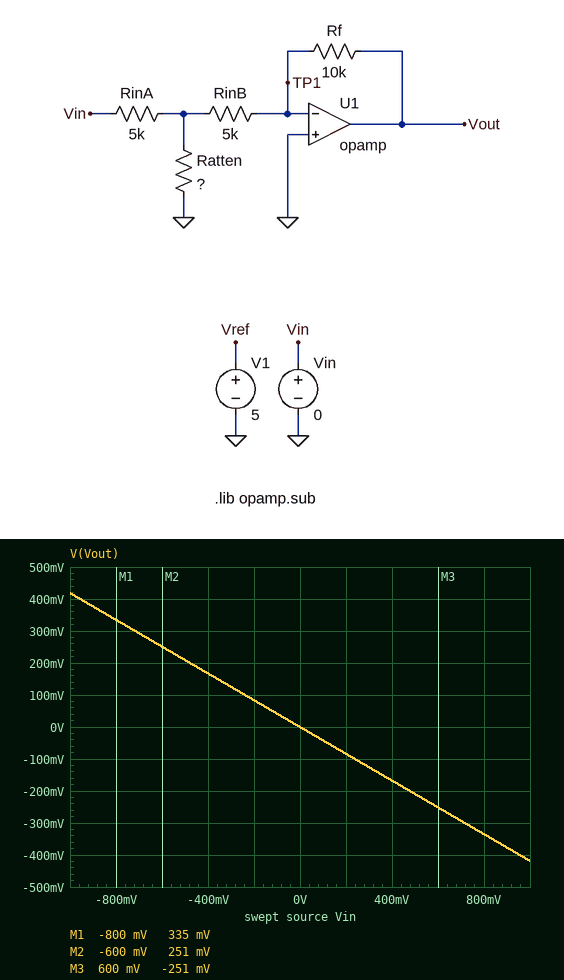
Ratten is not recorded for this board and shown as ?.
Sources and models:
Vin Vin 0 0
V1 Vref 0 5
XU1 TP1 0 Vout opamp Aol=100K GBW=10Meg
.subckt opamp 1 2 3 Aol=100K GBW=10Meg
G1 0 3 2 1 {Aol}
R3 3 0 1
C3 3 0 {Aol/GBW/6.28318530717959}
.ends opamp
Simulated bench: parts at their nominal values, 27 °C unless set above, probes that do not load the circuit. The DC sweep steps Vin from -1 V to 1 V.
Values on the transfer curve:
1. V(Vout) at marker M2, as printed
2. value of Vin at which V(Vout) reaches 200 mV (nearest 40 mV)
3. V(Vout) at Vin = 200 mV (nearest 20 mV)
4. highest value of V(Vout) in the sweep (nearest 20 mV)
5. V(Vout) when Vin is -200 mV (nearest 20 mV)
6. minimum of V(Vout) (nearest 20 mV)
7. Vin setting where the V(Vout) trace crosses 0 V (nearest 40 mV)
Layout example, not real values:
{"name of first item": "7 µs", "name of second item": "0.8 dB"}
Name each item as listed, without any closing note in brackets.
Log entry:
{"V(Vout) at marker M2, as printed": "251 mV", "value of Vin at which V(Vout) reaches 200 mV": "-480 mV", "V(Vout) at Vin = 200 mV": "-80 mV", "highest value of V(Vout) in the sweep": "420 mV", "V(Vout) when Vin is -200 mV": "80 mV", "minimum of V(Vout)": "-420 mV", "Vin setting where the V(Vout) trace crosses 0 V": "0 V"}
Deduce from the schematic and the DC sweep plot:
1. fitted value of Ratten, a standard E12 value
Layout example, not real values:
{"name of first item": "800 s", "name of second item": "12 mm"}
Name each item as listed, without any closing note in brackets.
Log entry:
{"fitted value of Ratten, a standard E12 value": "1.8 kΩ"}
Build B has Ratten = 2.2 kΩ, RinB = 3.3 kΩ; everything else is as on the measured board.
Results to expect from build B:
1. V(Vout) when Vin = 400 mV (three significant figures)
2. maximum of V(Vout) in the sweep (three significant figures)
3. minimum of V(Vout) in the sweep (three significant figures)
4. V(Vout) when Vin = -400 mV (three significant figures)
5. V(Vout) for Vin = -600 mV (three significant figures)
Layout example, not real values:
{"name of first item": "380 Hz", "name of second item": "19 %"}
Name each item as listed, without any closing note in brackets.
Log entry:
{"V(Vout) when Vin = 400 mV": "-253 mV", "maximum of V(Vout) in the sweep": "633 mV", "minimum of V(Vout) in the sweep": "-633 mV", "V(Vout) when Vin = -400 mV": "253 mV", "V(Vout) for Vin = -600 mV": "380 mV"}
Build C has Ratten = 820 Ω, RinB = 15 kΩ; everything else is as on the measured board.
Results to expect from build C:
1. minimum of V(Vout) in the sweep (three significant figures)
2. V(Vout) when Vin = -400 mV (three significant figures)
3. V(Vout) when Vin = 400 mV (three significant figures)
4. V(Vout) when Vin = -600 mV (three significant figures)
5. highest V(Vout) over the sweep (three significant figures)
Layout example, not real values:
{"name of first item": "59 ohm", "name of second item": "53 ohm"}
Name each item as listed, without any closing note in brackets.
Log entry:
{"minimum of V(Vout) in the sweep": "-89.7 mV", "V(Vout) when Vin = -400 mV": "35.9 mV", "V(Vout) when Vin = 400 mV": "-35.9 mV", "V(Vout) when Vin = -600 mV": "53.8 mV", "highest V(Vout) over the sweep": "89.7 mV"}
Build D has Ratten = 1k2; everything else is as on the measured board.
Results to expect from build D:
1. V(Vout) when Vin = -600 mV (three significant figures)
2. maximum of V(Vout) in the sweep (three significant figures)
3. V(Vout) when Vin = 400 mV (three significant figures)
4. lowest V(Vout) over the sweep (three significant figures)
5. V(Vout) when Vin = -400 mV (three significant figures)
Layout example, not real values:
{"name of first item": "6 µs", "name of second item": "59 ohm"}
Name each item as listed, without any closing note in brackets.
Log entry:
{"V(Vout) when Vin = -600 mV": "195 mV", "maximum of V(Vout) in the sweep": "324 mV", "V(Vout) when Vin = 400 mV": "-130 mV", "lowest V(Vout) over the sweep": "-324 mV", "V(Vout) when Vin = -400 mV": "130 mV"}
